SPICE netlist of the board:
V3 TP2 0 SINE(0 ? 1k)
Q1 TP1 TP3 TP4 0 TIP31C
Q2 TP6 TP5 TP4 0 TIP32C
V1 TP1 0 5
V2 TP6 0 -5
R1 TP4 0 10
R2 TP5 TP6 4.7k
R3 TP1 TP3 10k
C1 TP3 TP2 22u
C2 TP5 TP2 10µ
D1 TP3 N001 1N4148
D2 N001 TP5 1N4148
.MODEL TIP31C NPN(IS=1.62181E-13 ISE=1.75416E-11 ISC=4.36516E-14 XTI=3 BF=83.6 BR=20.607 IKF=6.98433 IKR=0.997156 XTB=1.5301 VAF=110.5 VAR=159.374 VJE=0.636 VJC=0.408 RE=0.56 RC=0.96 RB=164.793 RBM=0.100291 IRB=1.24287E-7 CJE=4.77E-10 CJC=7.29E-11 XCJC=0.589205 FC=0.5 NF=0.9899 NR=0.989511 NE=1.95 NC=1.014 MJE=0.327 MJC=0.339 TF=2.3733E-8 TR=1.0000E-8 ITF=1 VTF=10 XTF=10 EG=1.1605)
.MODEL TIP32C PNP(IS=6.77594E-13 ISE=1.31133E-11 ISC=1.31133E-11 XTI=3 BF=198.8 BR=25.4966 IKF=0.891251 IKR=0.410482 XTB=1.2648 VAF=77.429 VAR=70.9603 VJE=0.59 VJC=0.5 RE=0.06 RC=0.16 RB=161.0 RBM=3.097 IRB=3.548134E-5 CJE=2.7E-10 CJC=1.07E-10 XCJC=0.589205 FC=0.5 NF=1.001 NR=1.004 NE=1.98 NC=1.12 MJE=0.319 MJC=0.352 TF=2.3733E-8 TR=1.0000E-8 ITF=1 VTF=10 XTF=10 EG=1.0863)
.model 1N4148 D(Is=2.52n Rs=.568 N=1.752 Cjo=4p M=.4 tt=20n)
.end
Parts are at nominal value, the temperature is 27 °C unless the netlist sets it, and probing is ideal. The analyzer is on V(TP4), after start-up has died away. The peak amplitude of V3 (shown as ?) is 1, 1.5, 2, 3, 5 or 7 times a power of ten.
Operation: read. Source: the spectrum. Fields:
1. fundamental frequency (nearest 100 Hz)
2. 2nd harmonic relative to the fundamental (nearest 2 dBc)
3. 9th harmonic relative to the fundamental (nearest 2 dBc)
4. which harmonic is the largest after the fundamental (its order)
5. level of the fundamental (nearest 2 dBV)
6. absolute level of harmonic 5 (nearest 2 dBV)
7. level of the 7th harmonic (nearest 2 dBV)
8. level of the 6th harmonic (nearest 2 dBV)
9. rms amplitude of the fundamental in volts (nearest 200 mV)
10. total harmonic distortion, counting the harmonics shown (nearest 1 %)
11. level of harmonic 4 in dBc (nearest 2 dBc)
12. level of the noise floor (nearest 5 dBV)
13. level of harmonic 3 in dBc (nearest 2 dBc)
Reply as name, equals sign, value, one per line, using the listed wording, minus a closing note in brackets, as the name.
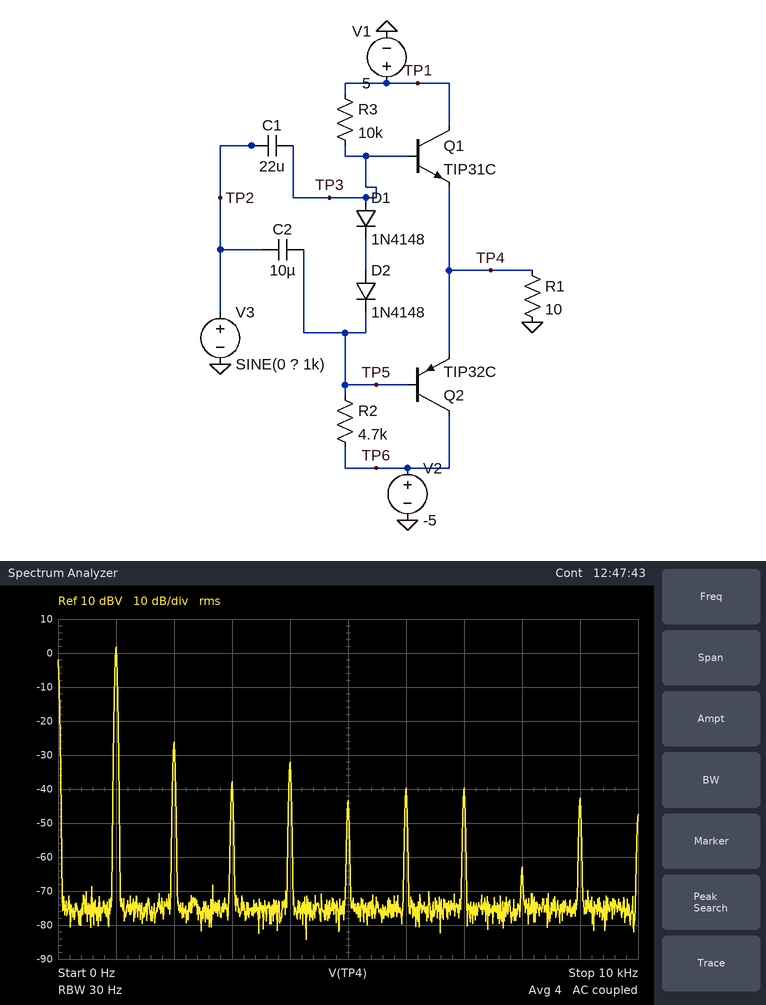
fundamental frequency = 1.0 kHz
2nd harmonic relative to the fundamental = -28 dBc
9th harmonic relative to the fundamental = -44 dBc
which harmonic is the largest after the fundamental = 2
level of the fundamental = 2 dBV
absolute level of harmonic 5 = -44 dBV
level of the 7th harmonic = -40 dBV
level of the 6th harmonic = -40 dBV
rms amplitude of the fundamental in volts = 1.2 V
total harmonic distortion, counting the harmonics shown = 5 %
level of harmonic 4 in dBc = -34 dBc
level of the noise floor = -75 dBV
level of harmonic 3 in dBc = -40 dBc
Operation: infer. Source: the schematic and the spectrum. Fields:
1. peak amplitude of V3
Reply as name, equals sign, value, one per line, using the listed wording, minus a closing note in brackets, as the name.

peak amplitude of V3 = 2 V
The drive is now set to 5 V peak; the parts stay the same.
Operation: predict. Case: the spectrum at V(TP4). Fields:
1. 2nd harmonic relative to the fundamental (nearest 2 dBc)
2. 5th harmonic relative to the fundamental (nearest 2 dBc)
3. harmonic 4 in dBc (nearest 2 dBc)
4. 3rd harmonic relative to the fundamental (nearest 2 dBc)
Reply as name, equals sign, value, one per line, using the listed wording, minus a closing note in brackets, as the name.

2nd harmonic relative to the fundamental = -20 dBc
5th harmonic relative to the fundamental = -30 dBc
harmonic 4 in dBc = -22 dBc
3rd harmonic relative to the fundamental = -18 dBc
